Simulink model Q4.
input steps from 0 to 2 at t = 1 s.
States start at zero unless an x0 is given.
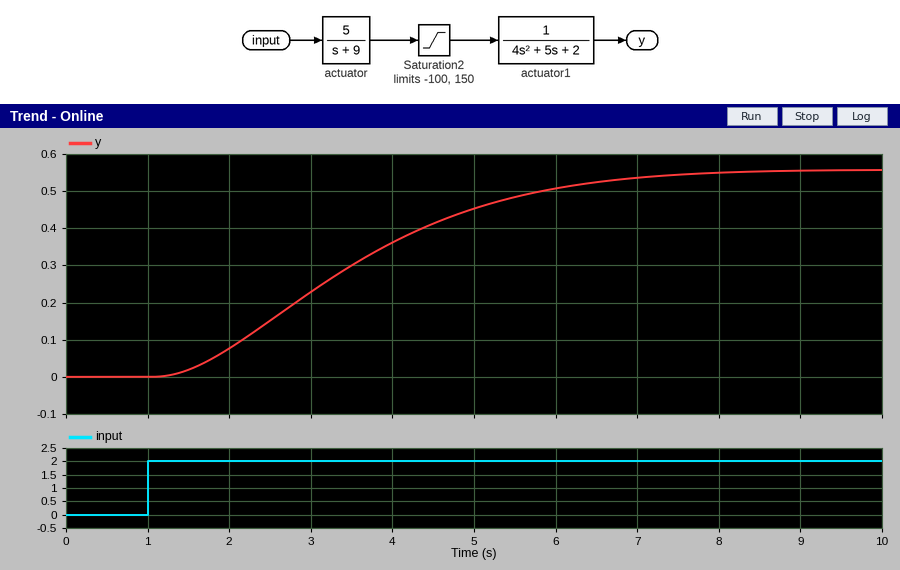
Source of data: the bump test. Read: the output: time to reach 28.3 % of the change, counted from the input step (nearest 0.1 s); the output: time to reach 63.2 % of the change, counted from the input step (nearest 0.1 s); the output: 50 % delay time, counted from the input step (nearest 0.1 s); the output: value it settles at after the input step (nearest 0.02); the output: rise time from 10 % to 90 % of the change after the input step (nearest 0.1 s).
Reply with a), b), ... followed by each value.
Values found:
a) 1.5 s
b) 2.9 s
c) 2.3 s
d) 0.56
e) 4.0 s
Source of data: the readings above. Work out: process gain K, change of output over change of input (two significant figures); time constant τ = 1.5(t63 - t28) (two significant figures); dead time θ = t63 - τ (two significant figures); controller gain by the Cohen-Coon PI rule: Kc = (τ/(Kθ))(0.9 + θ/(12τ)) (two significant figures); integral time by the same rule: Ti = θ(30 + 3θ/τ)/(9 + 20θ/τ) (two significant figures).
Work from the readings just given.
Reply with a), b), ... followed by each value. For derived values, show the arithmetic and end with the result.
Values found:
a) (0.56 - 0) / 2 = 0.28
b) 1.5 × (2.9 - 1.5) = 2.1 s
c) 2.9 - 2.1 = 0.80 s
d) 2.1 / (0.28 × 0.8) × (0.9 + 0.8 / (12 × 2.1)) = 8.7
e) 0.8 × (30 + 3 × 0.8 / 2.1) / (9 + 20 × 0.8 / 2.1) = 1.5 s
